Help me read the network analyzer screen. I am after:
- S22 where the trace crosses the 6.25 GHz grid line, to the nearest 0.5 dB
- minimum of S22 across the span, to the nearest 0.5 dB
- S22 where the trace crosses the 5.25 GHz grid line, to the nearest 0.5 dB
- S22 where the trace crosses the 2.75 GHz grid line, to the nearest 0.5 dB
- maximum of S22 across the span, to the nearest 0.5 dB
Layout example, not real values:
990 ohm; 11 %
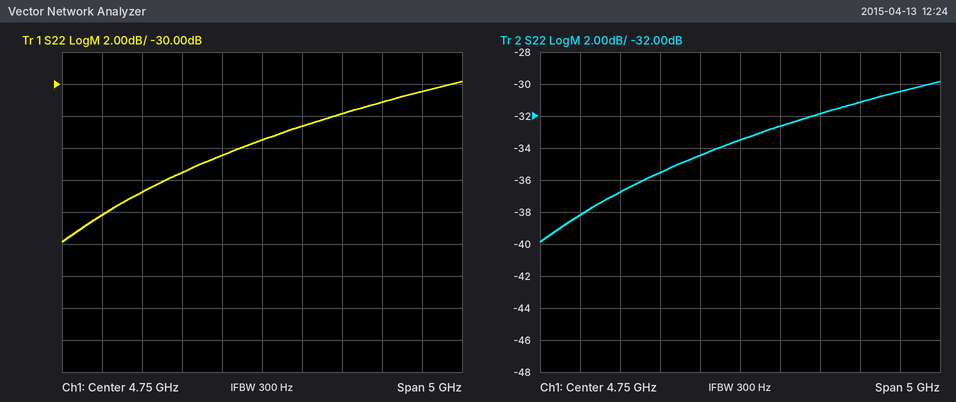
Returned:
-31.0 dB; -40.0 dB; -32.5 dB; -38.0 dB; -30.0 dB
